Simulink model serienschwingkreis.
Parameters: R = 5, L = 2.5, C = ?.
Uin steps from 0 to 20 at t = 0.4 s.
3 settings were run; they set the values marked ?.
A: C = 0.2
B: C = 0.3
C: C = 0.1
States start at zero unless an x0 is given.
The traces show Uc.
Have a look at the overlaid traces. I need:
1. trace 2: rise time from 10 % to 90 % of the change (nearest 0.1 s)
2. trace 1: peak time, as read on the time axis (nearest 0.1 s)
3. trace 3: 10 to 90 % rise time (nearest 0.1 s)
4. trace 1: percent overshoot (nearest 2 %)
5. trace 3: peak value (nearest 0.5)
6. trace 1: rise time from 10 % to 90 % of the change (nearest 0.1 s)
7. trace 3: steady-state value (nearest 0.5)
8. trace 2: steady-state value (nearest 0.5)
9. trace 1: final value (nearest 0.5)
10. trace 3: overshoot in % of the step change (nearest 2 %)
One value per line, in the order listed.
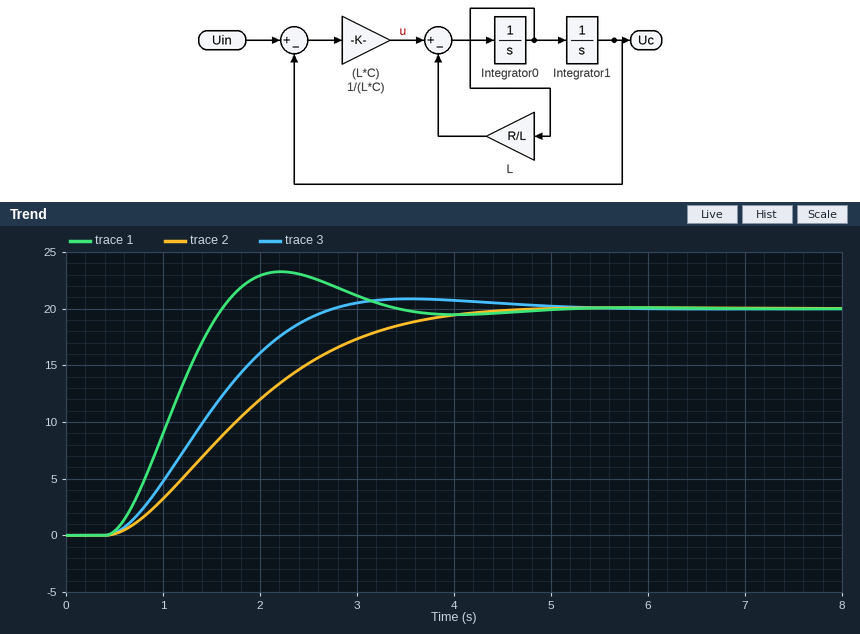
2.4 s
2.2 s
1.5 s
16 %
21.0
0.8 s
20.0
20.0
20.0
4 %
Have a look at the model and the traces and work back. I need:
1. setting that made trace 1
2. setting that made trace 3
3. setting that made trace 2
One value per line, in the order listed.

C
A
B
